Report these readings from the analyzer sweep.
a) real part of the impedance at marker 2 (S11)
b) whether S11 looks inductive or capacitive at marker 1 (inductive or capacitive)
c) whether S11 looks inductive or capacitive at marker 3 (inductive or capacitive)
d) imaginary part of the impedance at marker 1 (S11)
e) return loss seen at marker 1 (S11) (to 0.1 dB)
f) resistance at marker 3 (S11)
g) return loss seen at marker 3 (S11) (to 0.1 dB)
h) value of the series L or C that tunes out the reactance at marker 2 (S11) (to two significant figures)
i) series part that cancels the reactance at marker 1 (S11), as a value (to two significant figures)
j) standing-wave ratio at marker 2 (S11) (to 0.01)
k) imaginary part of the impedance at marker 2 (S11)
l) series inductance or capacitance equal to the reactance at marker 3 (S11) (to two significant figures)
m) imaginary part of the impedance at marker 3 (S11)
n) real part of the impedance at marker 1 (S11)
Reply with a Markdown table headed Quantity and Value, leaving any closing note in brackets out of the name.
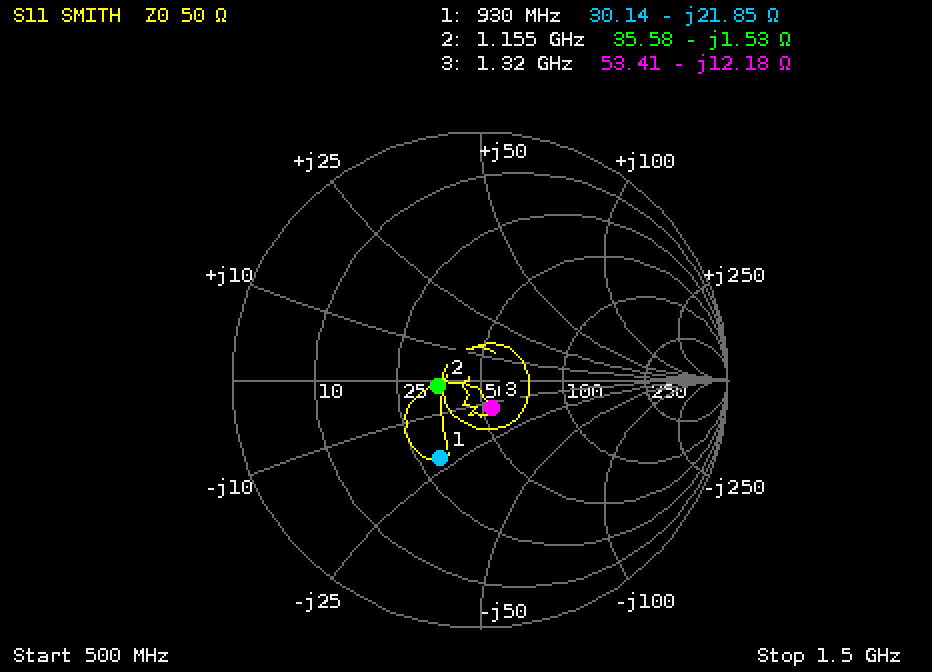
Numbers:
| Quantity | Value |
|---|---|
| real part of the impedance at marker 2 | 35.58 Ω |
| whether S11 looks inductive or capacitive at marker 1 | capacitive |
| whether S11 looks inductive or capacitive at marker 3 | capacitive |
| imaginary part of the impedance at marker 1 | -21.85 Ω |
| return loss seen at marker 1 (S11) | 9.0 dB |
| resistance at marker 3 | 53.41 Ω |
| return loss seen at marker 3 (S11) | 18.3 dB |
| value of the series L or C that tunes out the reactance at marker 2 (S11) | 210 pH |
| series part that cancels the reactance at marker 1 (S11), as a value | 3.7 nH |
| standing-wave ratio at marker 2 (S11) | 1.41 |
| imaginary part of the impedance at marker 2 | -1.53 Ω |
| series inductance or capacitance equal to the reactance at marker 3 (S11) | 9.9 pF |
| imaginary part of the impedance at marker 3 | -12.18 Ω |
| real part of the impedance at marker 1 | 30.14 Ω |
